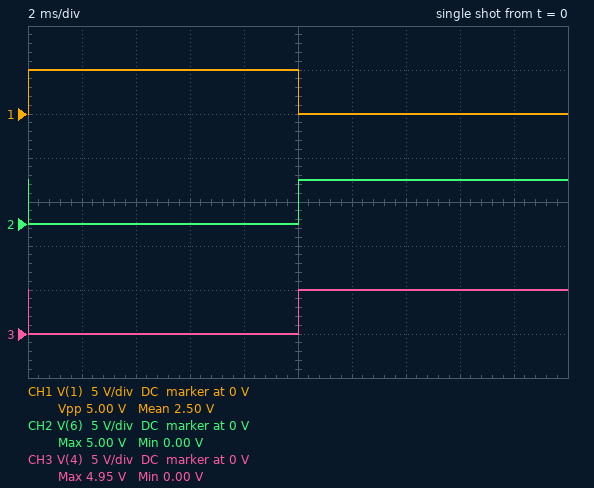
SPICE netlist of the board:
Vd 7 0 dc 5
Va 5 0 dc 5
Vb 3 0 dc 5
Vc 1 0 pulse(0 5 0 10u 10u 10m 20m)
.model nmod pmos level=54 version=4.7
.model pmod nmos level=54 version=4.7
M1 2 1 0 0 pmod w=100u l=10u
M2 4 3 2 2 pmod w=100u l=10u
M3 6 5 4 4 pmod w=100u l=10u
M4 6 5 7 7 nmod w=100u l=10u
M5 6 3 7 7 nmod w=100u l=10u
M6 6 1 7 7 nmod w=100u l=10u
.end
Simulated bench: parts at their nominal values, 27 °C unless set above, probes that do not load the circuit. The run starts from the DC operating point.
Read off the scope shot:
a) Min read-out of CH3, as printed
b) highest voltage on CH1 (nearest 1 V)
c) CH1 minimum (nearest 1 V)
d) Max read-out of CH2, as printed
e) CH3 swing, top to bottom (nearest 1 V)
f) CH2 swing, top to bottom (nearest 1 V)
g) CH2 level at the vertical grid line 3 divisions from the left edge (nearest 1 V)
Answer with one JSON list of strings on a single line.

["0.00 V", "5 V", "0 V", "5.00 V", "5 V", "5 V", "0 V"]
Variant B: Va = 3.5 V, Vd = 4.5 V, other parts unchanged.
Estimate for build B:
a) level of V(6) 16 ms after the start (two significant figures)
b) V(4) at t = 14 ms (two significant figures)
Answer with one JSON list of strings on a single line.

["4.5 V", "3.5 V"]
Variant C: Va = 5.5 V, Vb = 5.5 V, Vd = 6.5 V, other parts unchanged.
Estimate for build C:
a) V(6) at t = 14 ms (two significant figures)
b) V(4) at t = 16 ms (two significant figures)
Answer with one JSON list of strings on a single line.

["6.5 V", "5.5 V"]
